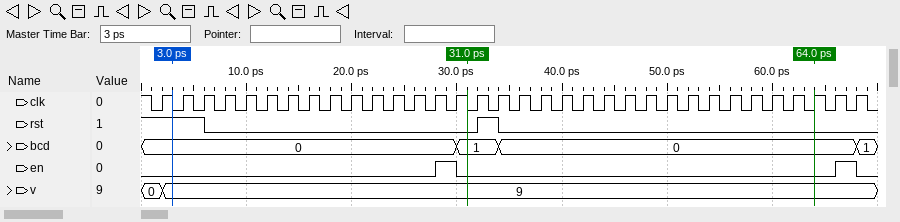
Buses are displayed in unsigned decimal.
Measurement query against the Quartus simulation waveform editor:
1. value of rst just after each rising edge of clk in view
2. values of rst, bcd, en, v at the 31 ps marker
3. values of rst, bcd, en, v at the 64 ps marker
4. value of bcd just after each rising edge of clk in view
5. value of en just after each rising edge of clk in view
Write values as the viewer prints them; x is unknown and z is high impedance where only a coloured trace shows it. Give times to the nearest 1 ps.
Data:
1 1 0 0 0 0 0 0 0 0 0 0 0 0 0 1 0 0 0 0 0 0 0 0 0 0 0 0 0 0 0 0 0 0
rst=0, bcd=1, en=0, v=9
rst=0, bcd=0, en=0, v=9
0, 0, 0, 0, 0, 0, 0, 0, 0, 0, 0, 0, 0, 0, 1, 1, 0, 0, 0, 0, 0, 0, 0, 0, 0, 0, 0, 0, 0, 0, 0, 0, 0, 1
0 0 0 0 0 0 0 0 0 0 0 0 0 1 0 0 0 0 0 0 0 0 0 0 0 0 0 0 0 0 0 0 1 0
